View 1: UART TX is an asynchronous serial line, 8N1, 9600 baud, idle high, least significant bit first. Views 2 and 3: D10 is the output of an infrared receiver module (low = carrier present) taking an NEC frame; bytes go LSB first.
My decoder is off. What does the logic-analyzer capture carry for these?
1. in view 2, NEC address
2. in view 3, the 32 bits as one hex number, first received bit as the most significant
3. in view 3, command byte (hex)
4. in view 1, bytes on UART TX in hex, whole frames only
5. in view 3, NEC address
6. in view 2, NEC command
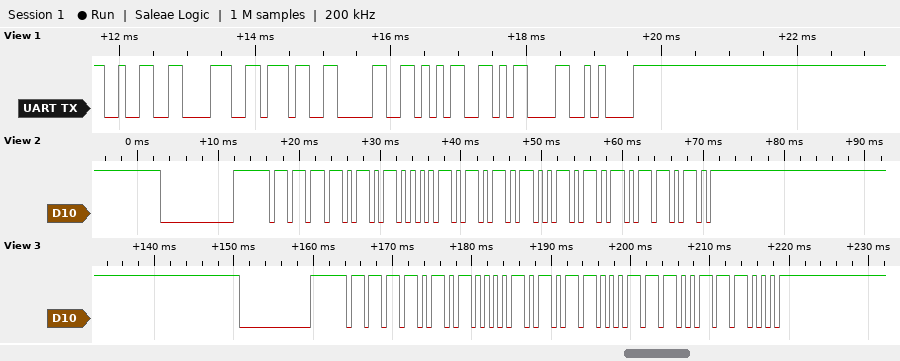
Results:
0xAF
0xF50AC738
0xE3
0x32 0x38 0x37 0x30 0x35 0x0D 0x0A
0xAF
0xA5
